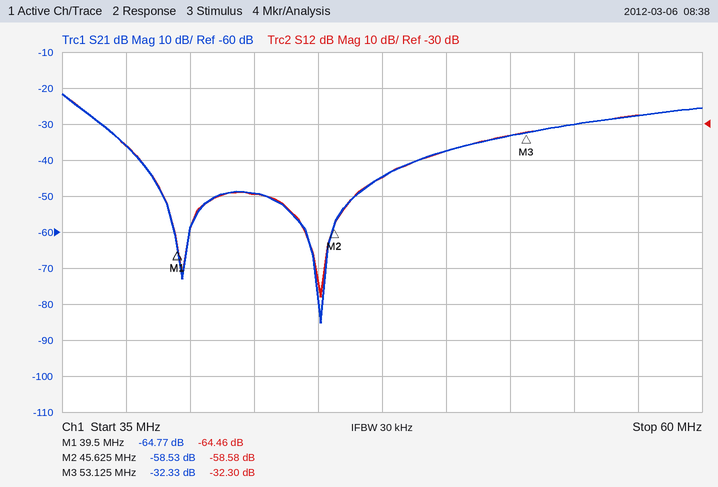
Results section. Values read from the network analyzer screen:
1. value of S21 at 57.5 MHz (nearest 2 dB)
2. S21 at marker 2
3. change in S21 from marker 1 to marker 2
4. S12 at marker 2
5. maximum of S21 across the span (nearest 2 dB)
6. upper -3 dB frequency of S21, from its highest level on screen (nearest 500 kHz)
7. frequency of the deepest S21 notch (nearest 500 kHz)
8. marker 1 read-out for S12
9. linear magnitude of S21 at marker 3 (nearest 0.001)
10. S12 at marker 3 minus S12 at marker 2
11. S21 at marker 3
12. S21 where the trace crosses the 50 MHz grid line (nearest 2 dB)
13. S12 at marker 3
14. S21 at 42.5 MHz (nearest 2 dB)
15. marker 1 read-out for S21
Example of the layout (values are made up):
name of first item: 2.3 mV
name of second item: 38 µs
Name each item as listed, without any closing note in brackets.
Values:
value of S21 at 57.5 MHz: -28 dB
S21 at marker 2: -58.53 dB
change in S21 from marker 1 to marker 2: 6.24 dB
S12 at marker 2: -58.58 dB
maximum of S21 across the span: -22 dB
upper -3 dB frequency of S21, from its highest level on screen: 35.5 MHz
frequency of the deepest S21 notch: 45.0 MHz
marker 1 read-out for S12: -64.46 dB
linear magnitude of S21 at marker 3: 0.024
S12 at marker 3 minus S12 at marker 2: 26.28 dB
S21 at marker 3: -32.33 dB
S21 where the trace crosses the 50 MHz grid line: -38 dB
S12 at marker 3: -32.30 dB
S21 at 42.5 MHz: -50 dB
marker 1 read-out for S21: -64.77 dB
